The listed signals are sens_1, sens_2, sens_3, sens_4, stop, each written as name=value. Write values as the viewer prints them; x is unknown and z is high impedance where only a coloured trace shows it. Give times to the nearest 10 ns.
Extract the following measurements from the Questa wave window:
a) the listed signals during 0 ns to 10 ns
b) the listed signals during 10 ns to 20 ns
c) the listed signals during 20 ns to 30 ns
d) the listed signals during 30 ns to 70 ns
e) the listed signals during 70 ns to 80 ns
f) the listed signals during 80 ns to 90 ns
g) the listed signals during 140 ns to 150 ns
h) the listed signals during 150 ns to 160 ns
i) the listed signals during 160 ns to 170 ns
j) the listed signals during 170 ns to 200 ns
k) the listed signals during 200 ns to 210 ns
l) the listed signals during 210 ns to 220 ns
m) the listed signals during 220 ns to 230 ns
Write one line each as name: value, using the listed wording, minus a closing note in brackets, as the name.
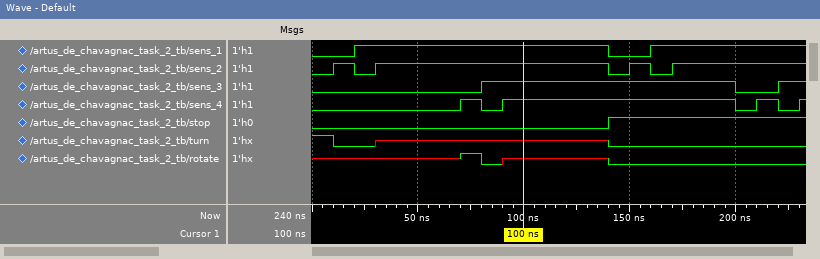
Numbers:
the listed signals during 0 ns to 10 ns: sens_1=0, sens_2=0, sens_3=0, sens_4=0, stop=0
the listed signals during 10 ns to 20 ns: sens_1=0, sens_2=1, sens_3=0, sens_4=0, stop=0
the listed signals during 20 ns to 30 ns: sens_1=1, sens_2=0, sens_3=0, sens_4=0, stop=0
the listed signals during 30 ns to 70 ns: sens_1=1, sens_2=1, sens_3=0, sens_4=0, stop=0
the listed signals during 70 ns to 80 ns: sens_1=1, sens_2=1, sens_3=0, sens_4=1, stop=0
the listed signals during 80 ns to 90 ns: sens_1=1, sens_2=1, sens_3=1, sens_4=0, stop=0
the listed signals during 140 ns to 150 ns: sens_1=0, sens_2=0, sens_3=1, sens_4=1, stop=1
the listed signals during 150 ns to 160 ns: sens_1=0, sens_2=1, sens_3=1, sens_4=1, stop=1
the listed signals during 160 ns to 170 ns: sens_1=1, sens_2=0, sens_3=1, sens_4=1, stop=1
the listed signals during 170 ns to 200 ns: sens_1=1, sens_2=1, sens_3=1, sens_4=1, stop=1
the listed signals during 200 ns to 210 ns: sens_1=1, sens_2=1, sens_3=0, sens_4=0, stop=1
the listed signals during 210 ns to 220 ns: sens_1=1, sens_2=1, sens_3=0, sens_4=1, stop=1
the listed signals during 220 ns to 230 ns: sens_1=1, sens_2=1, sens_3=1, sens_4=0, stop=1
